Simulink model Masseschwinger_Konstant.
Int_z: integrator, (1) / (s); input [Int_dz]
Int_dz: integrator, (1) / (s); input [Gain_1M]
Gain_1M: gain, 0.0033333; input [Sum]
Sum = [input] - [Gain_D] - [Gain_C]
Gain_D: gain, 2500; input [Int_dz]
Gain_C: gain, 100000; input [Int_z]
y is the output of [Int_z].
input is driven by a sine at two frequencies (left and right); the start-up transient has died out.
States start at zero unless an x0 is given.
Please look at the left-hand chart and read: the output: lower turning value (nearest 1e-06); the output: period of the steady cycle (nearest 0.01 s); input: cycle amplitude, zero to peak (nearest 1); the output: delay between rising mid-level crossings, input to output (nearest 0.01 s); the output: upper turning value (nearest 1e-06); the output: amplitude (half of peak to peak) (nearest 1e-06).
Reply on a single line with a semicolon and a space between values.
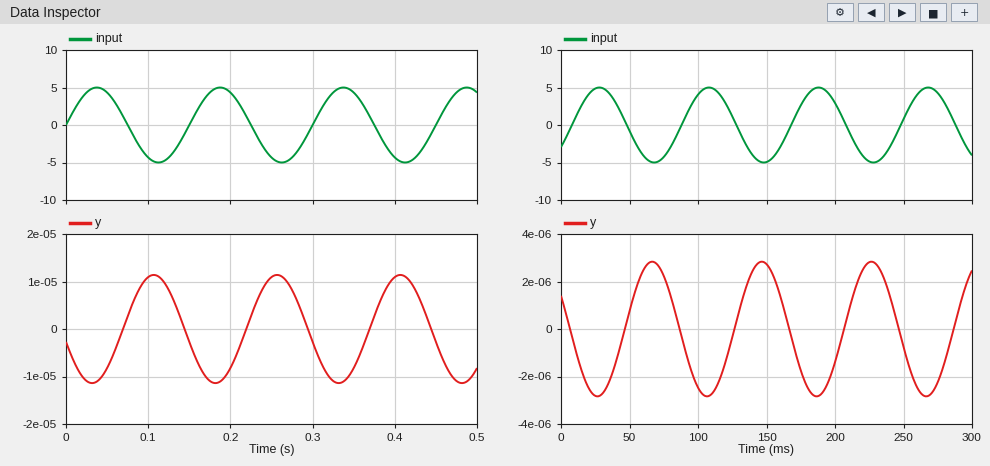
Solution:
-0.000011; 0.15 s; 5; 0.07 s; 0.000011; 0.000011
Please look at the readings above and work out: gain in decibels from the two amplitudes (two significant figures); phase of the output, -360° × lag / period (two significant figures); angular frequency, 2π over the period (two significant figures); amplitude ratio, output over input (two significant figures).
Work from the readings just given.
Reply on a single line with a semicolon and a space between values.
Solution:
-110 dB; -170°; 42 rad/s; 0.0000022
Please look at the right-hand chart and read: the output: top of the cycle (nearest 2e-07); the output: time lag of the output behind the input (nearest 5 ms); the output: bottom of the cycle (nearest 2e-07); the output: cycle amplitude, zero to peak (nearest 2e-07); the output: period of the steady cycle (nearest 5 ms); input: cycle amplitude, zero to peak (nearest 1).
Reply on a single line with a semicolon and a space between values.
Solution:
0.0000028; 40 ms; -0.0000028; 0.0000028; 80 ms; 5
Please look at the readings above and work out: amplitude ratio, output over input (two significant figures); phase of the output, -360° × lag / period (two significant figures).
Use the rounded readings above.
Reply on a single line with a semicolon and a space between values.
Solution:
0.00000056; -180°
